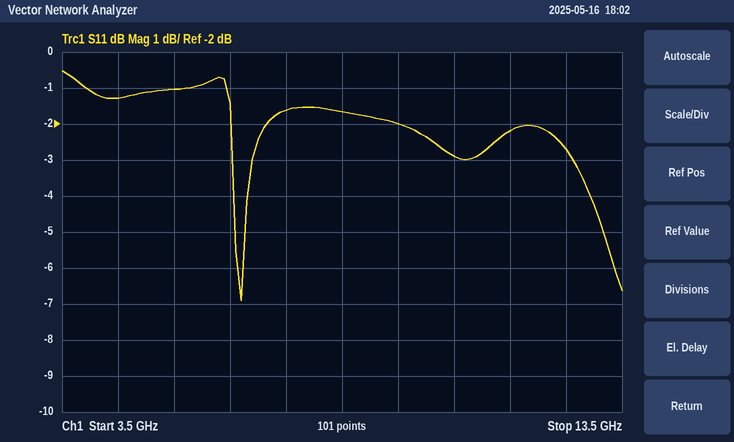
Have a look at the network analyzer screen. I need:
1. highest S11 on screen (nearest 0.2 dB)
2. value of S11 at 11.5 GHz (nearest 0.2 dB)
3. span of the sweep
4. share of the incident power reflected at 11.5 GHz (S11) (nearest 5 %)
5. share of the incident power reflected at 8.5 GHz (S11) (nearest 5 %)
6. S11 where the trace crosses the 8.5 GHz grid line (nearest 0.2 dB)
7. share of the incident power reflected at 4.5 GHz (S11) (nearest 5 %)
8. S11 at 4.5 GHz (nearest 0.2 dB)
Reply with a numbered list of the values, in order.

1. -0.6 dB
2. -2.2 dB
3. 10 GHz
4. 60 %
5. 70 %
6. -1.6 dB
7. 75 %
8. -1.2 dB
